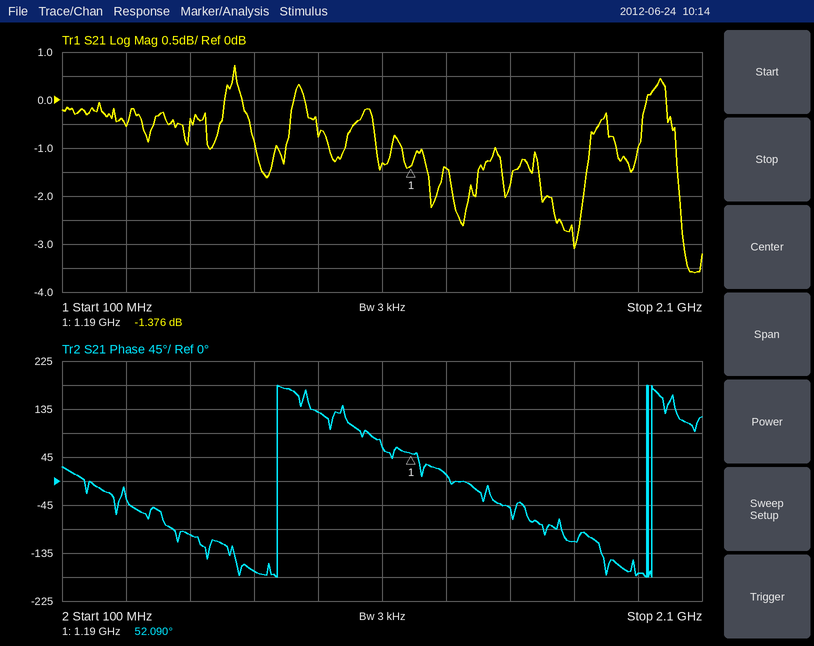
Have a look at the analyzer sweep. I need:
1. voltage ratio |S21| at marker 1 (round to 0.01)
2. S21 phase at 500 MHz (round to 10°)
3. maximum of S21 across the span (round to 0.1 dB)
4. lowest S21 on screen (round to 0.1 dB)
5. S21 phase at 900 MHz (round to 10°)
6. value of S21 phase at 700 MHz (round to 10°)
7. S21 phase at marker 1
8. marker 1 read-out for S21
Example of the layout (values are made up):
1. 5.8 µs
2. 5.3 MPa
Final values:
1. 0.85
2. -100°
3. 0.7 dB
4. -3.6 dB
5. 130°
6. -170°
7. 52.090°
8. -1.376 dB
